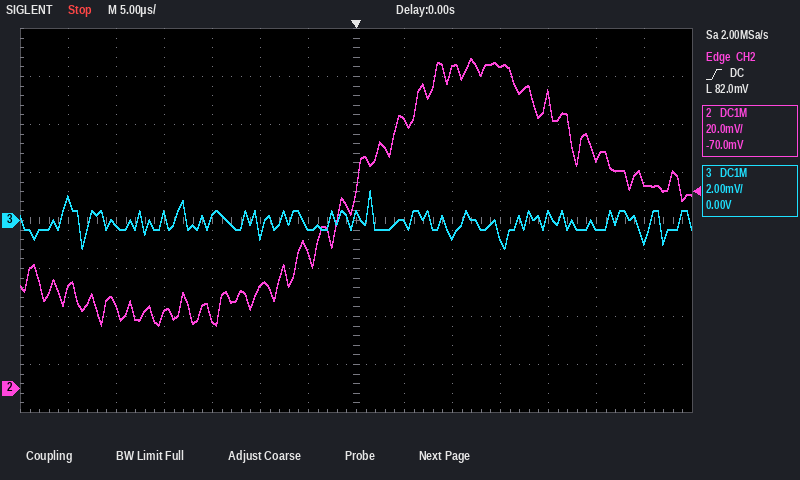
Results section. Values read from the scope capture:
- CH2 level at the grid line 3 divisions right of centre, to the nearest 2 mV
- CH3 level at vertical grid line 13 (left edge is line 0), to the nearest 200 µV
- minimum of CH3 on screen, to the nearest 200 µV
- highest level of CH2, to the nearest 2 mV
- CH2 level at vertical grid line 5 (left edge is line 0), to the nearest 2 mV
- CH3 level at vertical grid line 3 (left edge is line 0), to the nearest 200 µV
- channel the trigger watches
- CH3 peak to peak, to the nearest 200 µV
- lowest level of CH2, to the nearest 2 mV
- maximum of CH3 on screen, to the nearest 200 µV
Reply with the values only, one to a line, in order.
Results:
134 mV
-800 µV
-1.2 mV
138 mV
42 mV
200 µV
CH2
2.4 mV
26 mV
1.2 mV
